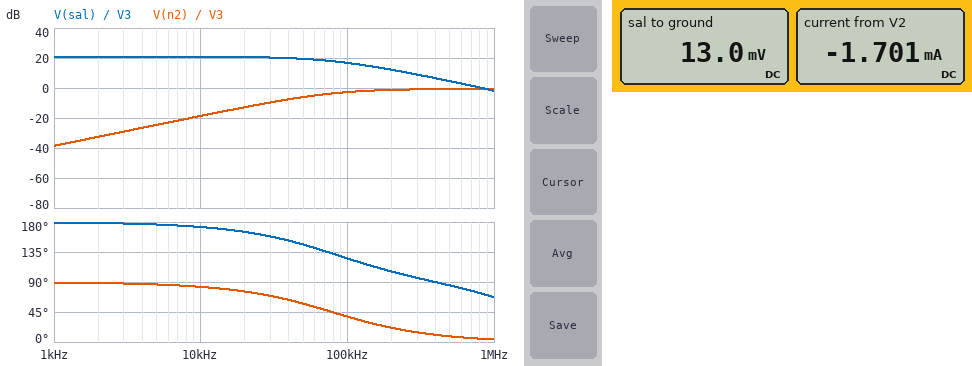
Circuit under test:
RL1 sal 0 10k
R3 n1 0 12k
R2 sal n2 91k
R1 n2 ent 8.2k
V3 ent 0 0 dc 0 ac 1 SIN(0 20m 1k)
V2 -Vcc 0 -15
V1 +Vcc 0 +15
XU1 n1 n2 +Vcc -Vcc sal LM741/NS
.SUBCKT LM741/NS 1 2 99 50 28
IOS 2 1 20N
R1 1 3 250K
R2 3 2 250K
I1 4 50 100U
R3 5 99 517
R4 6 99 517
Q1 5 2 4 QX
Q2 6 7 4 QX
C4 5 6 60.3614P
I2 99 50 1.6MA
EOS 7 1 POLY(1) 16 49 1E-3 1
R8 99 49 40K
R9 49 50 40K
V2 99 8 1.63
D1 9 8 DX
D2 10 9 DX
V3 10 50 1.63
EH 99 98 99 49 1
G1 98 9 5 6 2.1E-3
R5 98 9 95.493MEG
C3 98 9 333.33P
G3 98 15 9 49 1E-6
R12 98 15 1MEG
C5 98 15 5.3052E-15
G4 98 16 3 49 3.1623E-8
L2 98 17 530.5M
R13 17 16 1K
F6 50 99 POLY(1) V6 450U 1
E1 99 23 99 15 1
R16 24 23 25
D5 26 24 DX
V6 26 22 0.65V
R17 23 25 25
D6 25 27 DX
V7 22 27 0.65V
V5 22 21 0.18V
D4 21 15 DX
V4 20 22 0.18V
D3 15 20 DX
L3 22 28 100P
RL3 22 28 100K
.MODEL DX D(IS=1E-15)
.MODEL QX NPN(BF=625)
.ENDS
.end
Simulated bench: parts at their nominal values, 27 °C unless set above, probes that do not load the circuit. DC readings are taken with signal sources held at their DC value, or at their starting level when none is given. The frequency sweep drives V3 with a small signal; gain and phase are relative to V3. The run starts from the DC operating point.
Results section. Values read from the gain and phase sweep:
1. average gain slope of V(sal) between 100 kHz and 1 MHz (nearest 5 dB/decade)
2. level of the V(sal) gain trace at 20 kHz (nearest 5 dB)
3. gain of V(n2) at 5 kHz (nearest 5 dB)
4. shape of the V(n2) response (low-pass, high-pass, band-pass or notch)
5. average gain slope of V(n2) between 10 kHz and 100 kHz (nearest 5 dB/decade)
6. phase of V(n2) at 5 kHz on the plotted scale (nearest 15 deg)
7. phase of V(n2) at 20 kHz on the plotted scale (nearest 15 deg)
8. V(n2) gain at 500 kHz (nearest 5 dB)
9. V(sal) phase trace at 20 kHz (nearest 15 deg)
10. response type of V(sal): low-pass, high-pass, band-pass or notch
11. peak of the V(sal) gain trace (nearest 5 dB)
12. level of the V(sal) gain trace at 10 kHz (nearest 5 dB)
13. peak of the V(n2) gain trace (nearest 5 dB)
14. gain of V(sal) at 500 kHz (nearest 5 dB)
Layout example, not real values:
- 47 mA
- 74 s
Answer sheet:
- -20 dB/decade
- 20 dB
- -25 dB
- high-pass
- 15 dB/decade
- 90 deg
- 75 deg
- 0 dB
- 165 deg
- low-pass
- 20 dB
- 20 dB
- 0 dB
- 5 dB
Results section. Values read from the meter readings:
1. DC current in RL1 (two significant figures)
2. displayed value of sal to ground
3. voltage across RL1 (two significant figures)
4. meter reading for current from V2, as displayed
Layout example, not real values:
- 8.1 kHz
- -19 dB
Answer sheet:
- 1.3 µA
- 13.0 mV
- 13 mV
- -1.701 mA
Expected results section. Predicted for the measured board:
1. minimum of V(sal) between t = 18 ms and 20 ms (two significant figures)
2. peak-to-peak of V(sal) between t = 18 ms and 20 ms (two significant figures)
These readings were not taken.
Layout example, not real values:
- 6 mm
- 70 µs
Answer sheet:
- -210 mV
- 440 mV
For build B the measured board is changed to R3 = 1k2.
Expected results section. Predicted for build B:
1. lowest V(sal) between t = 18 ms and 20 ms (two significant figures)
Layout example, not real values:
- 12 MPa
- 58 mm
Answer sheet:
- -200 mV
